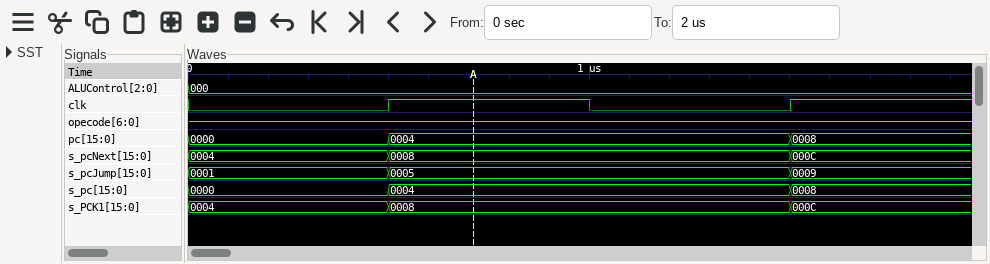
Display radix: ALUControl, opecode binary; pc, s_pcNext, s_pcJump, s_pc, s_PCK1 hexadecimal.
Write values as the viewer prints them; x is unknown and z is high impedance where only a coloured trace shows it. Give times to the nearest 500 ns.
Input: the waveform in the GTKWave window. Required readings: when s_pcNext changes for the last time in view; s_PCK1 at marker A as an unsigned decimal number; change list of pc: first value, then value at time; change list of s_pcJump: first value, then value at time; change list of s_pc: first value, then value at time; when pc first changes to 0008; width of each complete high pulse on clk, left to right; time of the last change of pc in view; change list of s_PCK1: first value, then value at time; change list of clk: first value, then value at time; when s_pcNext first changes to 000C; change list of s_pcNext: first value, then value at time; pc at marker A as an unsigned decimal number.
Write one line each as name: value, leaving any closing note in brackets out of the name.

when s_pcNext changes for the last time in view: 1500 ns
s_PCK1 at marker A as an unsigned decimal number: 8
change list of pc: first value, then value at time: 0000, 0004 at 500 ns, 0008 at 1500 ns
change list of s_pcJump: first value, then value at time: 0001, 0005 at 500 ns, 0009 at 1500 ns
change list of s_pc: first value, then value at time: 0000, 0004 at 500 ns, 0008 at 1500 ns
when pc first changes to 0008: 1500 ns
width of each complete high pulse on clk, left to right: 500 ns
time of the last change of pc in view: 1500 ns
change list of s_PCK1: first value, then value at time: 0004, 0008 at 500 ns, 000C at 1500 ns
change list of clk: first value, then value at time: 0, 1 at 500 ns, 0 at 1000 ns, 1 at 1500 ns
when s_pcNext first changes to 000C: 1500 ns
change list of s_pcNext: first value, then value at time: 0004, 0008 at 500 ns, 000C at 1500 ns
pc at marker A as an unsigned decimal number: 4
